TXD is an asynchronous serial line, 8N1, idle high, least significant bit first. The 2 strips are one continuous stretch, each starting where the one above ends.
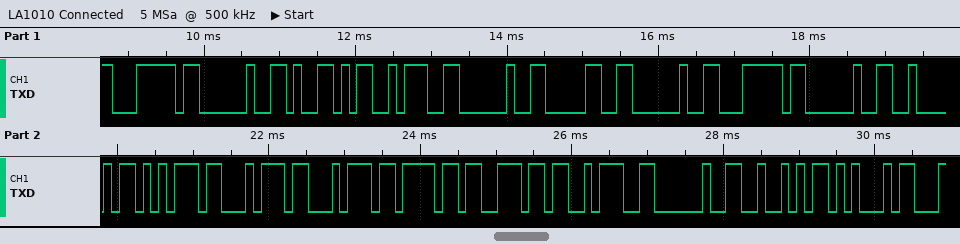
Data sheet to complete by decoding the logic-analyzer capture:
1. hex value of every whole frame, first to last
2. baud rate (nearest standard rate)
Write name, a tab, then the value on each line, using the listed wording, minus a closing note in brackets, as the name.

hex value of every whole frame, first to last	7C 20 59 3A 20 30 20 7C 20 42 75 74 74 6F 6E 3A 20 52 45
baud rate	9600 baud
